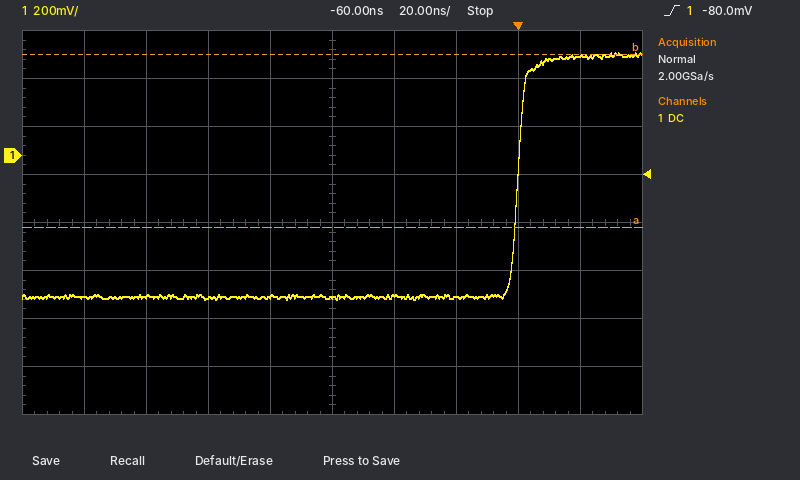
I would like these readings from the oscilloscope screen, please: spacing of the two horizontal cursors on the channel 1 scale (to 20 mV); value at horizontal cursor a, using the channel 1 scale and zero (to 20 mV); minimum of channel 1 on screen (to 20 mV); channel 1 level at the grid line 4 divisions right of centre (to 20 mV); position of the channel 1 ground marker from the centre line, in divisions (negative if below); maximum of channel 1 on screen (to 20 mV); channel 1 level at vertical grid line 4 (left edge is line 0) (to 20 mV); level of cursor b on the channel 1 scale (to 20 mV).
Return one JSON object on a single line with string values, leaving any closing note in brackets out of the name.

{"spacing of the two horizontal cursors on the channel 1 scale": "720 mV", "value at horizontal cursor a, using the channel 1 scale and zero": "-300 mV", "minimum of channel 1 on screen": "-600 mV", "channel 1 level at the grid line 4 divisions right of centre": "420 mV", "position of the channel 1 ground marker from the centre line, in divisions": "+1.4 div", "maximum of channel 1 on screen": "420 mV", "channel 1 level at vertical grid line 4 (left edge is line 0)": "-580 mV", "level of cursor b on the channel 1 scale": "420 mV"}
